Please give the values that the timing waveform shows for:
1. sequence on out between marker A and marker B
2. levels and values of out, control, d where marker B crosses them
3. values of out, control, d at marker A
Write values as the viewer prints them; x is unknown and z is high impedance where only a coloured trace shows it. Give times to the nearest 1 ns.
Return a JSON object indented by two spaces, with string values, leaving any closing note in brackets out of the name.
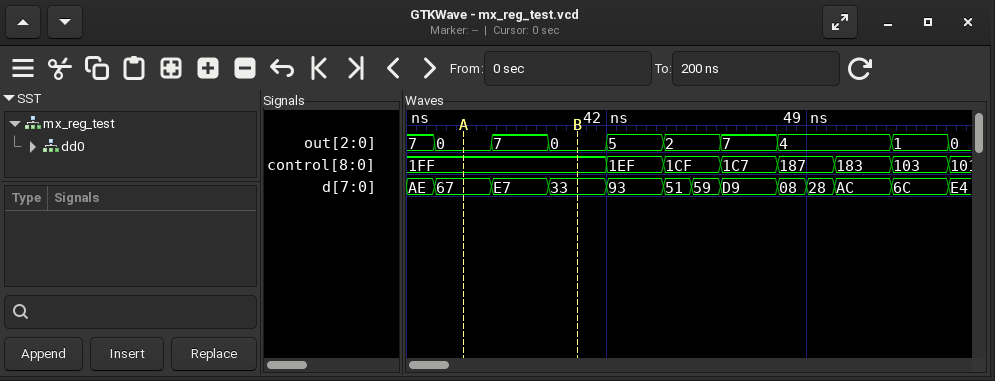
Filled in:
{
  "sequence on out between marker A and marker B": "0, 7, 0",
  "levels and values of out, control, d where marker B crosses them": "out=0, control=1FF, d=33",
  "values of out, control, d at marker A": "out=0, control=1FF, d=67"
}
